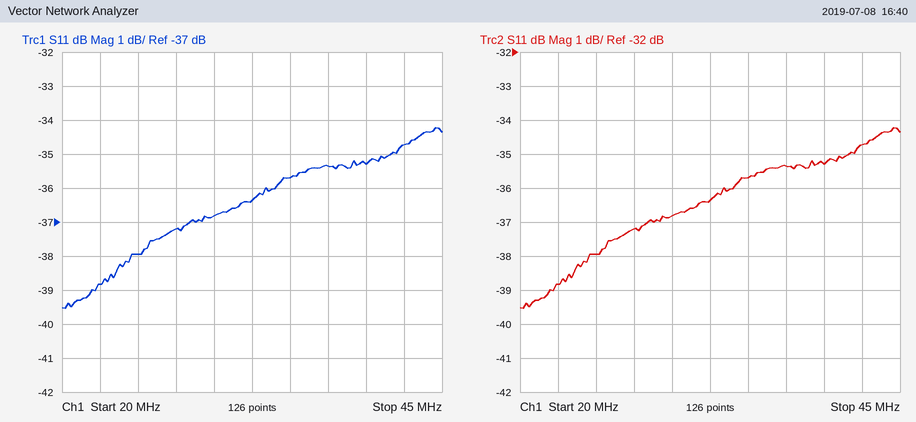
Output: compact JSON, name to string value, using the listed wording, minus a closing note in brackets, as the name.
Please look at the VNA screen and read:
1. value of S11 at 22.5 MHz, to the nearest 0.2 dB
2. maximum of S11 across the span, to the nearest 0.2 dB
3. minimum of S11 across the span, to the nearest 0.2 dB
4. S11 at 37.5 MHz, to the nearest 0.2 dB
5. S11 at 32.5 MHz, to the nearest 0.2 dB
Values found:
{"value of S11 at 22.5 MHz, to the nearest 0.2 dB": "-38.8 dB", "maximum of S11 across the span, to the nearest 0.2 dB": "-34.2 dB", "minimum of S11 across the span, to the nearest 0.2 dB": "-39.6 dB", "S11 at 37.5 MHz, to the nearest 0.2 dB": "-35.4 dB", "S11 at 32.5 MHz, to the nearest 0.2 dB": "-36.4 dB"}
